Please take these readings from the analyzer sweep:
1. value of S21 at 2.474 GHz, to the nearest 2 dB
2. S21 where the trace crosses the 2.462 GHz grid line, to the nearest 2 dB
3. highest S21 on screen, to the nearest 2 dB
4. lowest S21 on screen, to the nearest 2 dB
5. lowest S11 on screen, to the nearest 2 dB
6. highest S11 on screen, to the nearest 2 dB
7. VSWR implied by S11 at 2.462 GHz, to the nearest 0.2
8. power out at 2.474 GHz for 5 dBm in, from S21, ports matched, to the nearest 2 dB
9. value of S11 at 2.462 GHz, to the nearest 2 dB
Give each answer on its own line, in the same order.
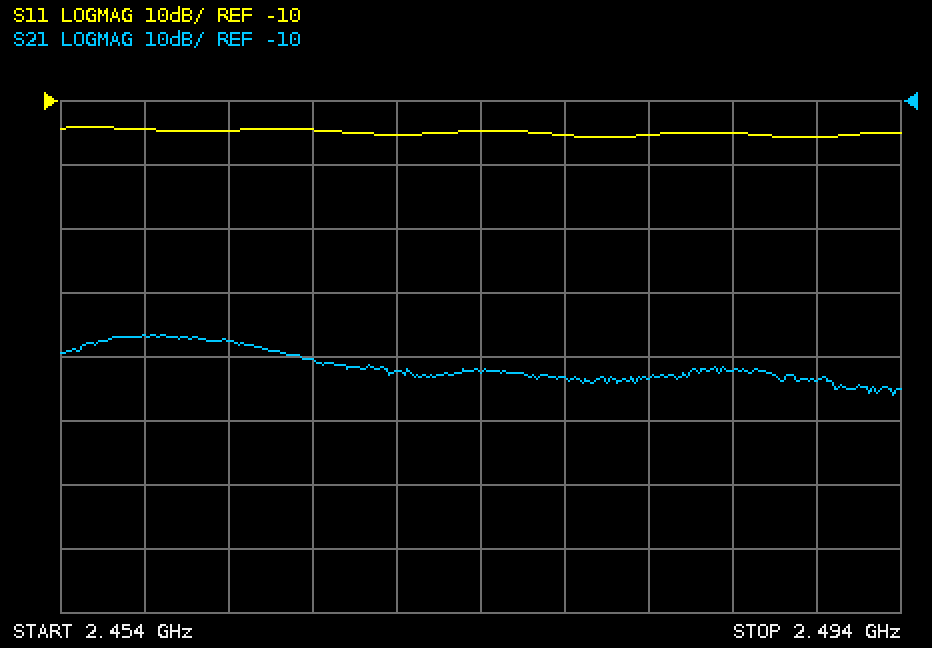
-52 dB
-48 dB
-46 dB
-56 dB
-16 dB
-14 dB
1.4
-48 dBm
-14 dB
